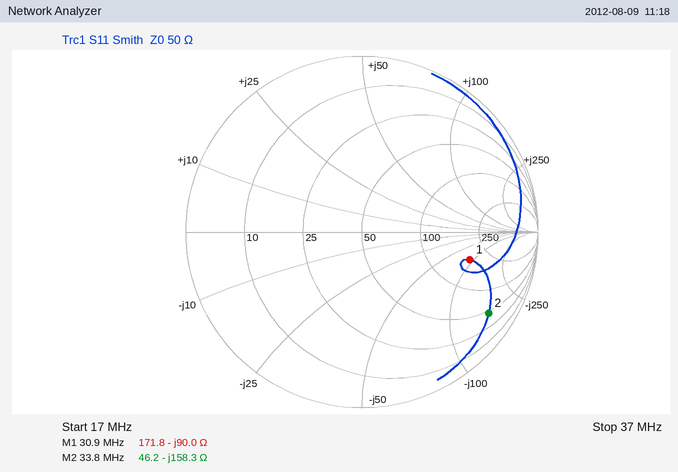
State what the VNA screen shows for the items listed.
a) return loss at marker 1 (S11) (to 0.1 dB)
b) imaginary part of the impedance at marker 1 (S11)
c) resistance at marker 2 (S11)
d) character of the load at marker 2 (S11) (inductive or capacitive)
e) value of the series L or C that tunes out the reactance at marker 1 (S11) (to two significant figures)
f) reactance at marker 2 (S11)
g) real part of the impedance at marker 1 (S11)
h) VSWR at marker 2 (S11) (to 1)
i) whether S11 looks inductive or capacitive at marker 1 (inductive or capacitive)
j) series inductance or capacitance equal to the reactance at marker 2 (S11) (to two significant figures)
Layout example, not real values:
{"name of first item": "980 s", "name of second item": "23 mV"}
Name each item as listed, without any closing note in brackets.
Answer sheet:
{"return loss at marker 1 (S11)": "4.0 dB", "imaginary part of the impedance at marker 1": "-90.0 Ω", "resistance at marker 2": "46.2 Ω", "character of the load at marker 2 (S11)": "capacitive", "value of the series L or C that tunes out the reactance at marker 1 (S11)": "460 nH", "reactance at marker 2": "-158.3 Ω", "real part of the impedance at marker 1": "171.8 Ω", "VSWR at marker 2 (S11)": "13", "whether S11 looks inductive or capacitive at marker 1": "capacitive", "series inductance or capacitance equal to the reactance at marker 2 (S11)": "30 pF"}
